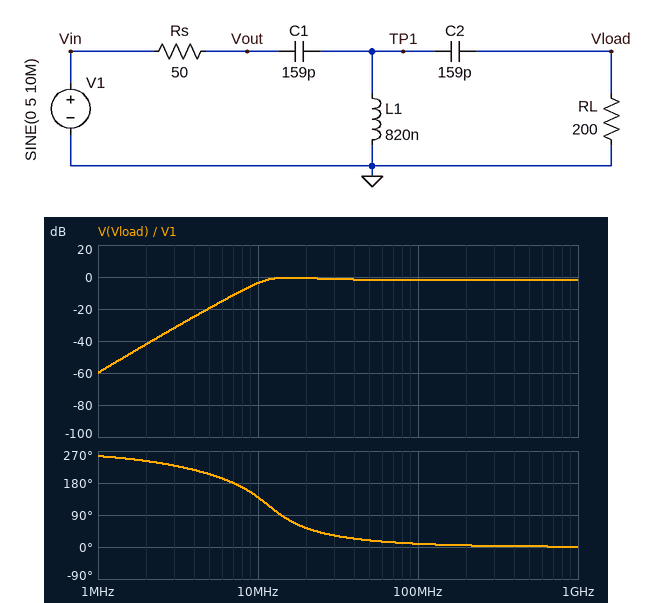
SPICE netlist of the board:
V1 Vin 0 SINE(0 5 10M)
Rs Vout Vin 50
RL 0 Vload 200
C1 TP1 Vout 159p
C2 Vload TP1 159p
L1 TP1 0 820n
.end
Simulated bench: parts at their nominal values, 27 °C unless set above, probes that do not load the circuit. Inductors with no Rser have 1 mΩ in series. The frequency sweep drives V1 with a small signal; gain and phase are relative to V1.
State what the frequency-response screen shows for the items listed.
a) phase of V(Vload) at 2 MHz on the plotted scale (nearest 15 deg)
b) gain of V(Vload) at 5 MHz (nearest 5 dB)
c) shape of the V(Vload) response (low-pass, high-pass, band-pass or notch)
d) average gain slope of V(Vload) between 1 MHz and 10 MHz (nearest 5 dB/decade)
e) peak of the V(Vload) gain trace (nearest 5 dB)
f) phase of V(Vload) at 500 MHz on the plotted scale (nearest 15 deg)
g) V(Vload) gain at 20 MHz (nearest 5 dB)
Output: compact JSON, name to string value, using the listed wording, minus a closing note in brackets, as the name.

{"phase of V(Vload) at 2 MHz on the plotted scale": "240 deg", "gain of V(Vload) at 5 MHz": "-20 dB", "shape of the V(Vload) response": "high-pass", "average gain slope of V(Vload) between 1 MHz and 10 MHz": "55 dB/decade", "peak of the V(Vload) gain trace": "0 dB", "phase of V(Vload) at 500 MHz on the plotted scale": "0 deg", "V(Vload) gain at 20 MHz": "0 dB"}
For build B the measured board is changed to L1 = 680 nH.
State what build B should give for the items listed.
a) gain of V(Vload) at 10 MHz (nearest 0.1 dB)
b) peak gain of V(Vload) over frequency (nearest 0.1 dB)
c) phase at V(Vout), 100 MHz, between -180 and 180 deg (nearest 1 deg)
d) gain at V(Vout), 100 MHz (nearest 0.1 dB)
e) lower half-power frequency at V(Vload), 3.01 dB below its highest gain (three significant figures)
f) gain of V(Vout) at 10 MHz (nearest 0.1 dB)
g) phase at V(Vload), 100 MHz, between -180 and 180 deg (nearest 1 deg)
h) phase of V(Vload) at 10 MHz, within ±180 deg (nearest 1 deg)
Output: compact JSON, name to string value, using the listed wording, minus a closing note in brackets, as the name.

{"gain of V(Vload) at 10 MHz": "-5.8 dB", "peak gain of V(Vload) over frequency": "-0.5 dB", "phase at V(Vout), 100 MHz, between -180 and 180 deg": "4 deg", "gain at V(Vout), 100 MHz": "-2.0 dB", "lower half-power frequency at V(Vload), 3.01 dB below its highest gain": "11.4 MHz", "gain of V(Vout) at 10 MHz": "-3.2 dB", "phase at V(Vload), 100 MHz, between -180 and 180 deg": "10 deg", "phase of V(Vload) at 10 MHz, within ±180 deg": "149 deg"}
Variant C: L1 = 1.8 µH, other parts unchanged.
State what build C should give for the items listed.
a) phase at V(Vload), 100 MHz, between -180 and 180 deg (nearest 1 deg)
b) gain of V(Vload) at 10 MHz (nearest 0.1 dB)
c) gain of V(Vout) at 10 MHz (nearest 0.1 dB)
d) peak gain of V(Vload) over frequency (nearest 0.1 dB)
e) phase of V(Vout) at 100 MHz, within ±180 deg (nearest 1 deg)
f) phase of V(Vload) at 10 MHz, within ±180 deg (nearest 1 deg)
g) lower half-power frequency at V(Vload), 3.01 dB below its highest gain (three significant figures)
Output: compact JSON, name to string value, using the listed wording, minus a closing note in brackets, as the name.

{"phase at V(Vload), 100 MHz, between -180 and 180 deg": "7 deg", "gain of V(Vload) at 10 MHz": "-0.1 dB", "gain of V(Vout) at 10 MHz": "-5.0 dB", "peak gain of V(Vload) over frequency": "0 dB", "phase of V(Vout) at 100 MHz, within ±180 deg": "1 deg", "phase of V(Vload) at 10 MHz, within ±180 deg": "82 deg", "lower half-power frequency at V(Vload), 3.01 dB below its highest gain": "6.65 MHz"}
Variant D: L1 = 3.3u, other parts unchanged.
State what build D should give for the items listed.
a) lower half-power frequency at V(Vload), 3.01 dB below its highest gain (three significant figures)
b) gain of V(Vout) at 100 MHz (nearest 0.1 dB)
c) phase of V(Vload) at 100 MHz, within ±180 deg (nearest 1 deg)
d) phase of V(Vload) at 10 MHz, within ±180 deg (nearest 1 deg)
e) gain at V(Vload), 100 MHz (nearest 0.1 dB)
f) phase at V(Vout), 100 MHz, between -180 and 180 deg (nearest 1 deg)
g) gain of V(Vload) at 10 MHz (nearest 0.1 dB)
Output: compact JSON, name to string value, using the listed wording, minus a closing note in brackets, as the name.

{"lower half-power frequency at V(Vload), 3.01 dB below its highest gain": "4.75 MHz", "gain of V(Vout) at 100 MHz": "-1.9 dB", "phase of V(Vload) at 100 MHz, within ±180 deg": "6 deg", "phase of V(Vload) at 10 MHz, within ±180 deg": "57 deg", "gain at V(Vload), 100 MHz": "-1.9 dB", "phase at V(Vout), 100 MHz, between -180 and 180 deg": "0 deg", "gain of V(Vload) at 10 MHz": "-1.5 dB"}
